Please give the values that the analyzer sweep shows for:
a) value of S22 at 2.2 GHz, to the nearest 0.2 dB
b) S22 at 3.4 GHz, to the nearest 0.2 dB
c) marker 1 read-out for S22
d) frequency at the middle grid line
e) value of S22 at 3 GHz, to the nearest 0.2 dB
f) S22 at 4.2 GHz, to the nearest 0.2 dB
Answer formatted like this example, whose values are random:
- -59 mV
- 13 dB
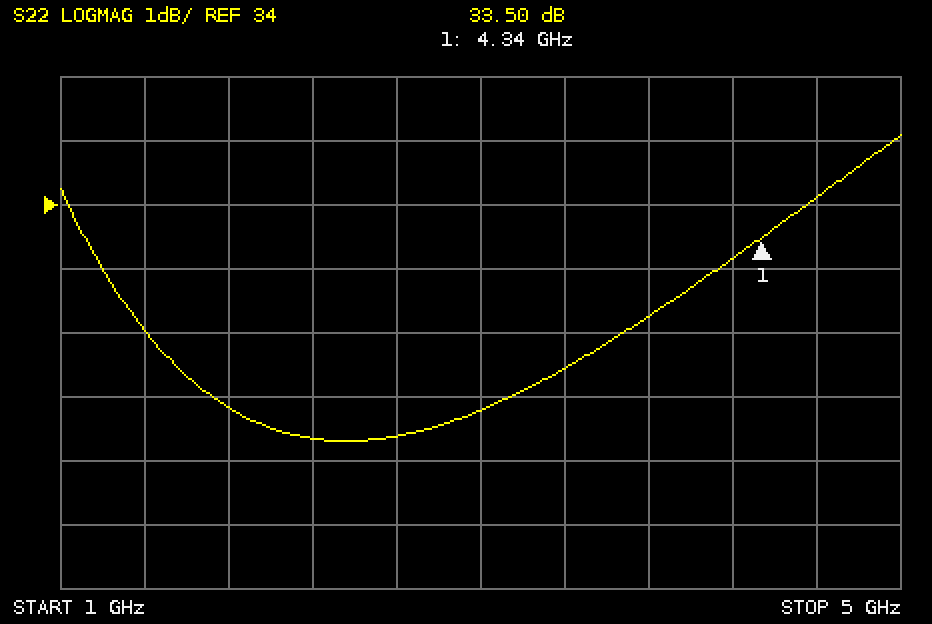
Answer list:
- 30.4 dB
- 31.4 dB
- 33.50 dB
- 3 GHz
- 30.8 dB
- 33.2 dB
